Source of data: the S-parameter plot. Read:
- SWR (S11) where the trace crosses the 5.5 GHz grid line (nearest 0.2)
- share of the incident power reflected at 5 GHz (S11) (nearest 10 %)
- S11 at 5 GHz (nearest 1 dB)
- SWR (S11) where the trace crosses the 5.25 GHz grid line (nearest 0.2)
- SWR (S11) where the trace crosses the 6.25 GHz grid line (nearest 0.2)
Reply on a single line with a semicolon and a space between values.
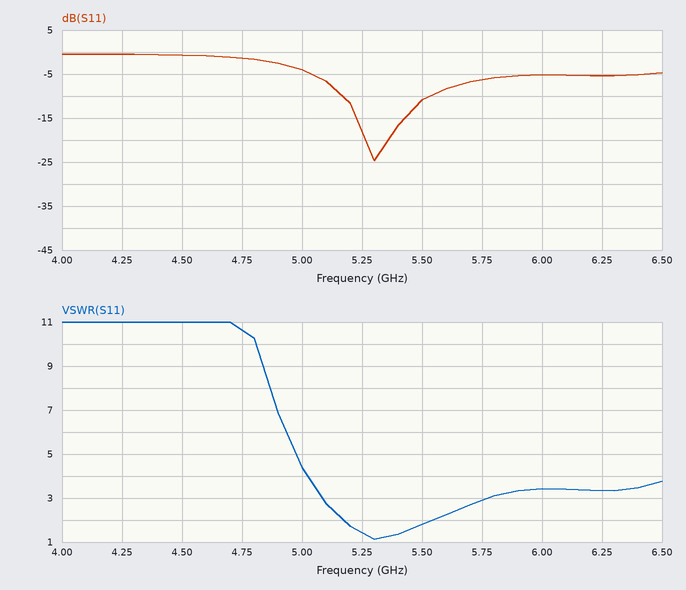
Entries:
1.8; 40 %; -4 dB; 1.4; 3.4
